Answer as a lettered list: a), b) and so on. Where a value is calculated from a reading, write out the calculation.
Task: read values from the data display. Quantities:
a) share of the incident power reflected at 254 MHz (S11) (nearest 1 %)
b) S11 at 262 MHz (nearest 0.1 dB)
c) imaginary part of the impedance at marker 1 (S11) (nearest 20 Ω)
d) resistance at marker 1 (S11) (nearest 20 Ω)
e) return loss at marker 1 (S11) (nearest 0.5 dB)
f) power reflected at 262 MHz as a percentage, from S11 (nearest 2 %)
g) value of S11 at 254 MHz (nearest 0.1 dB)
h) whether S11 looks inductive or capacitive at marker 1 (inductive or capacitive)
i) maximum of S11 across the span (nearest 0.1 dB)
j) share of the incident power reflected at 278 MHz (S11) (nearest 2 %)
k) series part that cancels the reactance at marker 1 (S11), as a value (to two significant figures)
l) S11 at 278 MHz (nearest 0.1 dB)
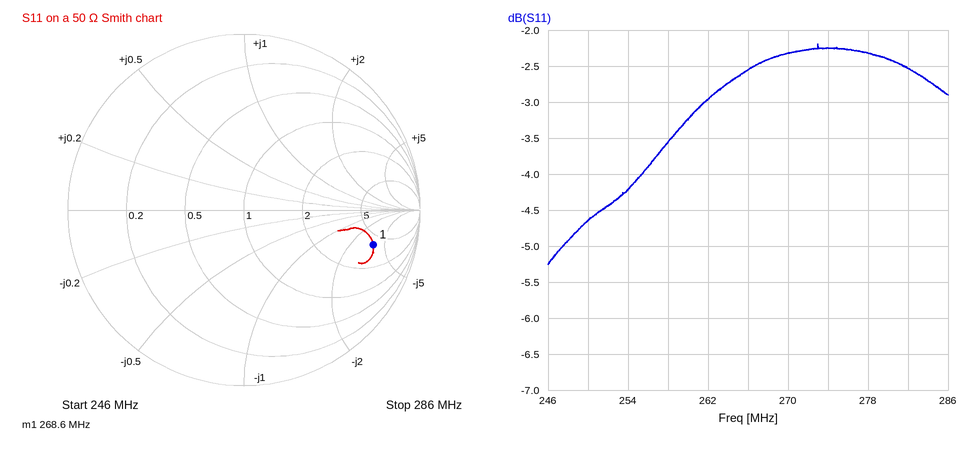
a) 10^(-4.2/10) ≈ 38 %
b) -3.0 dB
c) -180 Ω
d) 200 Ω
e) 2.5 dB
f) 10^(-3/10) ≈ 50 %
g) -4.2 dB
h) capacitive
i) -2.2 dB
j) 10^(-2.3/10) ≈ 58.9 %, so 58 % to the nearest 2 %
k) L = 180 Ω/(2π × 268.6 MHz) ≈ 107 nH, so 110 nH to two significant figures
l) -2.3 dB
